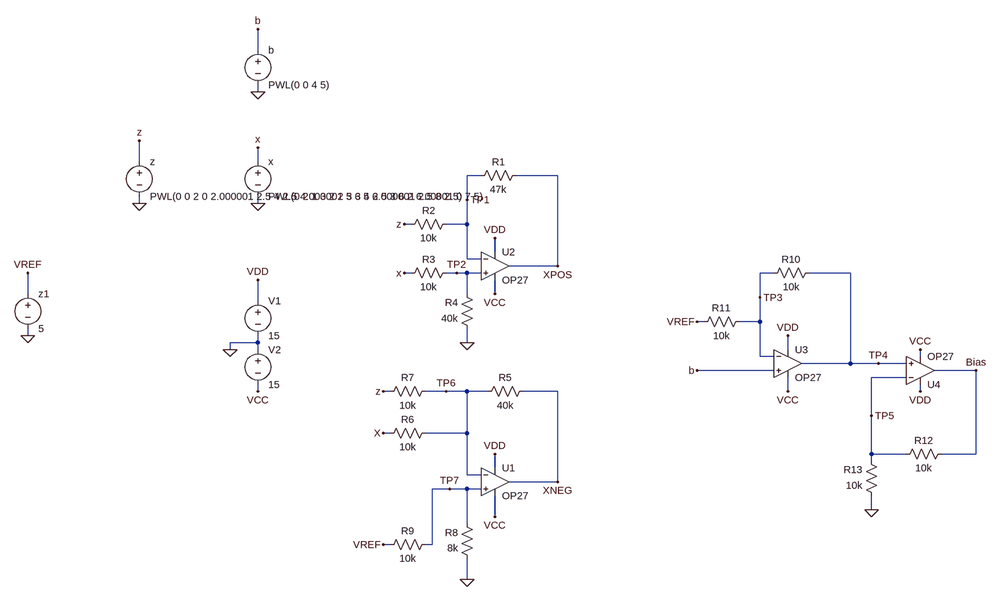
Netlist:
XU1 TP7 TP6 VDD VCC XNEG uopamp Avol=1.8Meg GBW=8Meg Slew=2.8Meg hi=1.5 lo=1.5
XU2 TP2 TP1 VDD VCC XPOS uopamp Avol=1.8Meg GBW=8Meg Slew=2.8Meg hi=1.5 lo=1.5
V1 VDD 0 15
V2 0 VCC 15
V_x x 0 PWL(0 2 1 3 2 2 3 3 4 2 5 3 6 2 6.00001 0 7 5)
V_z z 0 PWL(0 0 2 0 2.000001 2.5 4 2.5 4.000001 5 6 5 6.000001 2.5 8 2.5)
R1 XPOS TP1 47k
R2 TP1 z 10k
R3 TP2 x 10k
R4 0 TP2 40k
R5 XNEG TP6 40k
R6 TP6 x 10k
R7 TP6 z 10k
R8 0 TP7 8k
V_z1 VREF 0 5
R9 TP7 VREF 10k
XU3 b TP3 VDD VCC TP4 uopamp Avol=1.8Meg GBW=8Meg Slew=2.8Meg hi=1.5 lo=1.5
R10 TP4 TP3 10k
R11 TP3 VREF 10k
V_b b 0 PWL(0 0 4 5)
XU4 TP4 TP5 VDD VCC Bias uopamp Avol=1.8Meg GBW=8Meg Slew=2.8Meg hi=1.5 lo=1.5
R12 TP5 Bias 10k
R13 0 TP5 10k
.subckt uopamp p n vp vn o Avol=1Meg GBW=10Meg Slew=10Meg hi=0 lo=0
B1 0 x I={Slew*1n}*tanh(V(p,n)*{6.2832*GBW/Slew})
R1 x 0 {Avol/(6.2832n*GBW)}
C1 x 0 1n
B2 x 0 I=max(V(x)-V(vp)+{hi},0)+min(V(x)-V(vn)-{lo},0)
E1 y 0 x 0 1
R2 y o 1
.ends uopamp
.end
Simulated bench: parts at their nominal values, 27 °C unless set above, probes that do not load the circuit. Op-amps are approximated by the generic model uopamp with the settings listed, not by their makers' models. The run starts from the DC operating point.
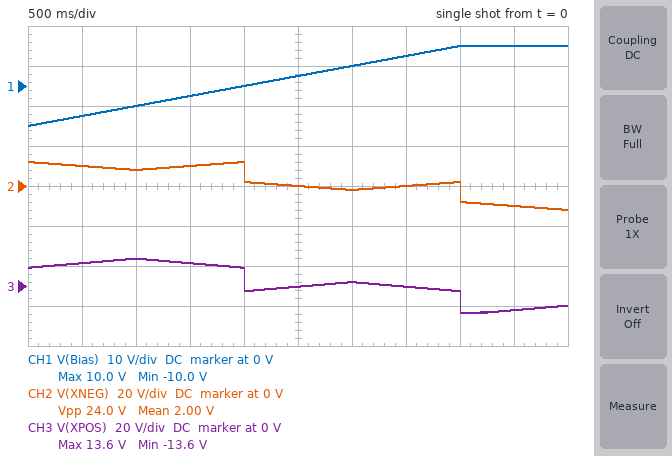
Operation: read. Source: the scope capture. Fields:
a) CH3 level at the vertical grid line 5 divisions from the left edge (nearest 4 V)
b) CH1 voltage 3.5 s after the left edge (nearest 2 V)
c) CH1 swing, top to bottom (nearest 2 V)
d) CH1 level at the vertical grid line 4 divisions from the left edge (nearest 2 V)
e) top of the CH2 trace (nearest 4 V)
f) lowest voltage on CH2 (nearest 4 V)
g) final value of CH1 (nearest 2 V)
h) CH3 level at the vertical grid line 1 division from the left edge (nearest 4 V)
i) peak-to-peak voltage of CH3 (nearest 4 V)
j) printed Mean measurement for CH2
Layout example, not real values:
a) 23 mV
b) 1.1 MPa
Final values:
a) 0 V
b) 8 V
c) 20 V
d) 0 V
e) 12 V
f) -12 V
g) 10 V
h) 12 V
i) 28 V
j) 2.00 V
